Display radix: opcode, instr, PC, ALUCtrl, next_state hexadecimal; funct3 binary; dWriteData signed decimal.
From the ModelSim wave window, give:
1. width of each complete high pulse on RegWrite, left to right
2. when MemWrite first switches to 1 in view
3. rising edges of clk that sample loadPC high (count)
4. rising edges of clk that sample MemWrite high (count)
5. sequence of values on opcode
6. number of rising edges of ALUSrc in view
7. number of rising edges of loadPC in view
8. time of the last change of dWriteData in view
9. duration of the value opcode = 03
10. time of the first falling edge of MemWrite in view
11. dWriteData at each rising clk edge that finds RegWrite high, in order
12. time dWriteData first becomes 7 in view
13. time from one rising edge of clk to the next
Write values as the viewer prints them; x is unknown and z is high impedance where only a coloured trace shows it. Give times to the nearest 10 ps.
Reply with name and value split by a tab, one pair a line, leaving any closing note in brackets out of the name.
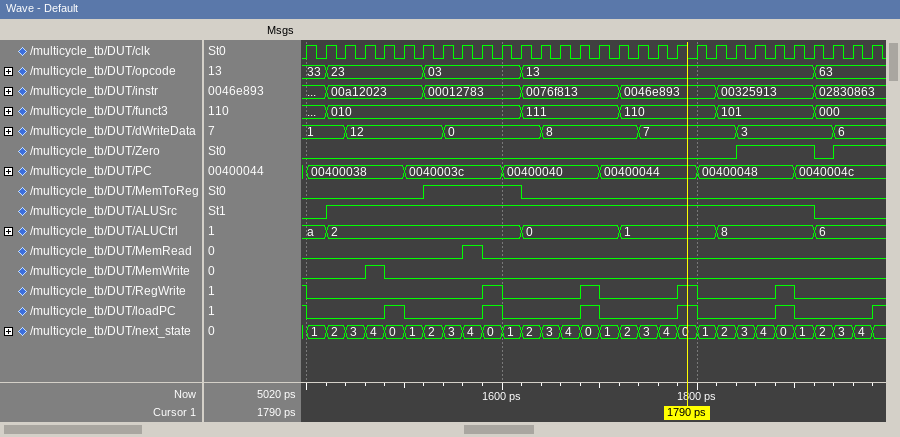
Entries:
width of each complete high pulse on RegWrite, left to right	20 ps, 20 ps, 20 ps, 20 ps
when MemWrite first switches to 1 in view	1460 ps
rising edges of clk that sample loadPC high	6
rising edges of clk that sample MemWrite high	1
sequence of values on opcode	33, 23, 03, 13, 63
number of rising edges of ALUSrc in view	1
number of rising edges of loadPC in view	6
time of the last change of dWriteData in view	1940 ps
duration of the value opcode = 03	100 ps
time of the first falling edge of MemWrite in view	1480 ps
dWriteData at each rising clk edge that finds RegWrite high, in order	1, 0, 8, 7, 3
time dWriteData first becomes 7 in view	1740 ps
time from one rising edge of clk to the next	20 ps
